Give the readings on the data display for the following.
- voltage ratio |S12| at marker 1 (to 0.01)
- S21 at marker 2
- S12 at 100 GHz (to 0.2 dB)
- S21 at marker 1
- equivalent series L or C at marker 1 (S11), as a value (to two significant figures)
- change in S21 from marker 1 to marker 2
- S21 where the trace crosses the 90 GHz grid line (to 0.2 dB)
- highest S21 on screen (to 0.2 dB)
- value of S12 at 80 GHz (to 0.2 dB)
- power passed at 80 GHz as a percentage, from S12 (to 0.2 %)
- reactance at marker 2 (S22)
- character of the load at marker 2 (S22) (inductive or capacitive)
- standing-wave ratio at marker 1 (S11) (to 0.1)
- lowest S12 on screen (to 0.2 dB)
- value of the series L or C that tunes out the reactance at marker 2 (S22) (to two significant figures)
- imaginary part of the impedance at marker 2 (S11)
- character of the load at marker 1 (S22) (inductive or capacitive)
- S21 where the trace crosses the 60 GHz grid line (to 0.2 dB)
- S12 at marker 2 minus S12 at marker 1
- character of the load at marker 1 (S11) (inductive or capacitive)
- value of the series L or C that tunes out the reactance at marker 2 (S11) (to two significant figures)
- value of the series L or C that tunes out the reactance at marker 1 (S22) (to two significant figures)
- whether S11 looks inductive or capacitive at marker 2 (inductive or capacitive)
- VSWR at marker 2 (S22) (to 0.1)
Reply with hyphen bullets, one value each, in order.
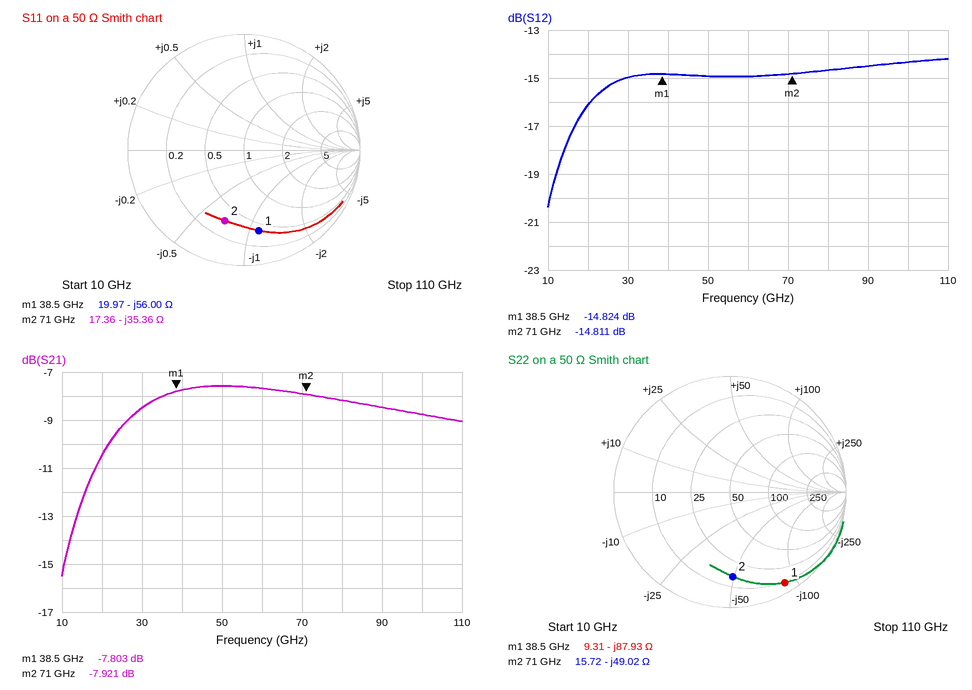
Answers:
- 0.18
- -7.921 dB
- -14.4 dB
- -7.803 dB
- 74 fF
- -0.118 dB
- -8.4 dB
- -7.6 dB
- -14.6 dB
- 3.4 %
- -49.02 Ω
- capacitive
- 5.9
- -20.4 dB
- 110 pH
- -35.36 Ω
- capacitive
- -7.6 dB
- 0.013 dB
- capacitive
- 79 pH
- 360 pH
- capacitive
- 6.4
